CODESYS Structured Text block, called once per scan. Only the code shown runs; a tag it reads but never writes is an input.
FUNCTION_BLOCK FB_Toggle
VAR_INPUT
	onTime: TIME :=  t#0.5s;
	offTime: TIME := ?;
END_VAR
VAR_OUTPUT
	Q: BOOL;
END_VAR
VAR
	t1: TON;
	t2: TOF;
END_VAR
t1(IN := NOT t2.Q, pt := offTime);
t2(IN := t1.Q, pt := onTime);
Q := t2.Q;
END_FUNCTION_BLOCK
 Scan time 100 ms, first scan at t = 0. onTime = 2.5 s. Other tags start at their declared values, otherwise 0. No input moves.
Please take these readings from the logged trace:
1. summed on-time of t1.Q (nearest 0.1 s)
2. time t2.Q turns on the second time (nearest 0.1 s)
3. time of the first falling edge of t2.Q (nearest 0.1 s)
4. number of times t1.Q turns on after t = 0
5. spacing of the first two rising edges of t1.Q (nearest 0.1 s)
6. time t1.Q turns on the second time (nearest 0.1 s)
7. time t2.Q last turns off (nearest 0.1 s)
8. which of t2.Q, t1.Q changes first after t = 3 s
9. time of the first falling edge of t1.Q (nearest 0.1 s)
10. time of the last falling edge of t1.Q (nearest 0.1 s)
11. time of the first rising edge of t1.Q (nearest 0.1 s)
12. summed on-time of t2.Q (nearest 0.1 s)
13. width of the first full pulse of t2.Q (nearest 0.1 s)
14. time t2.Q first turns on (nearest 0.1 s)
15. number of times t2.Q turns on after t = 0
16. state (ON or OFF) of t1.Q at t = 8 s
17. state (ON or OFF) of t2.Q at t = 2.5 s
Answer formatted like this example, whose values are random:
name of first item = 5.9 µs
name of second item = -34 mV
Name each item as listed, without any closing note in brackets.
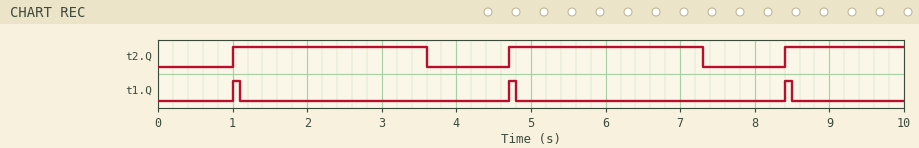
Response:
summed on-time of t1.Q = 0.3 s
time t2.Q turns on the second time = 4.7 s
time of the first falling edge of t2.Q = 3.6 s
number of times t1.Q turns on after t = 0 = 3
spacing of the first two rising edges of t1.Q = 3.7 s
time t1.Q turns on the second time = 4.7 s
time t2.Q last turns off = 7.3 s
which of t2.Q, t1.Q changes first after t = 3 s = t2.Q
time of the first falling edge of t1.Q = 1.1 s
time of the last falling edge of t1.Q = 8.5 s
time of the first rising edge of t1.Q = 1.0 s
summed on-time of t2.Q = 6.8 s
width of the first full pulse of t2.Q = 2.6 s
time t2.Q first turns on = 1.0 s
number of times t2.Q turns on after t = 0 = 3
state (ON or OFF) of t1.Q at t = 8 s = OFF
state (ON or OFF) of t2.Q at t = 2.5 s = ON
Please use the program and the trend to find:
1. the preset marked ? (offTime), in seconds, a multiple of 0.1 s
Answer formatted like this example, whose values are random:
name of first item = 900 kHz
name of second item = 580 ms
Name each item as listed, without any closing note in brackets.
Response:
the preset marked ? (offTime), in seconds, a multiple of 0.1 s = 1.0 s
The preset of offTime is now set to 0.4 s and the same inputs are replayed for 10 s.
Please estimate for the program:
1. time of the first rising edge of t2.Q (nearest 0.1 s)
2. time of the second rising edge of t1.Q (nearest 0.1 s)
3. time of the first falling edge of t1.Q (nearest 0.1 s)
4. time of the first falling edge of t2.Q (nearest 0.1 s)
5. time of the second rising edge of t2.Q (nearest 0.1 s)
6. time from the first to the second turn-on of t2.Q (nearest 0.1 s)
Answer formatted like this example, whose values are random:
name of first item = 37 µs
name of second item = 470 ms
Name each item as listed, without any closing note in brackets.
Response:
time of the first rising edge of t2.Q = 0.4 s
time of the second rising edge of t1.Q = 3.5 s
time of the first falling edge of t1.Q = 0.5 s
time of the first falling edge of t2.Q = 3.0 s
time of the second rising edge of t2.Q = 3.5 s
time from the first to the second turn-on of t2.Q = 3.1 s
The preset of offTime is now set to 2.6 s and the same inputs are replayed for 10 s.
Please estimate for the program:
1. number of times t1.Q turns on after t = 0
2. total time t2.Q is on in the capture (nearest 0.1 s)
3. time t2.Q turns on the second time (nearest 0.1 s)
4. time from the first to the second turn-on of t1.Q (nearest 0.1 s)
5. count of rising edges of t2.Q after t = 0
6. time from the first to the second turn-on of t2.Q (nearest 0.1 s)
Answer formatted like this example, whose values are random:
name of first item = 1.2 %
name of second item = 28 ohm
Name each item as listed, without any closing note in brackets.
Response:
number of times t1.Q turns on after t = 0 = 2
total time t2.Q is on in the capture = 4.7 s
time t2.Q turns on the second time = 7.9 s
time from the first to the second turn-on of t1.Q = 5.3 s
count of rising edges of t2.Q after t = 0 = 2
time from the first to the second turn-on of t2.Q = 5.3 s
